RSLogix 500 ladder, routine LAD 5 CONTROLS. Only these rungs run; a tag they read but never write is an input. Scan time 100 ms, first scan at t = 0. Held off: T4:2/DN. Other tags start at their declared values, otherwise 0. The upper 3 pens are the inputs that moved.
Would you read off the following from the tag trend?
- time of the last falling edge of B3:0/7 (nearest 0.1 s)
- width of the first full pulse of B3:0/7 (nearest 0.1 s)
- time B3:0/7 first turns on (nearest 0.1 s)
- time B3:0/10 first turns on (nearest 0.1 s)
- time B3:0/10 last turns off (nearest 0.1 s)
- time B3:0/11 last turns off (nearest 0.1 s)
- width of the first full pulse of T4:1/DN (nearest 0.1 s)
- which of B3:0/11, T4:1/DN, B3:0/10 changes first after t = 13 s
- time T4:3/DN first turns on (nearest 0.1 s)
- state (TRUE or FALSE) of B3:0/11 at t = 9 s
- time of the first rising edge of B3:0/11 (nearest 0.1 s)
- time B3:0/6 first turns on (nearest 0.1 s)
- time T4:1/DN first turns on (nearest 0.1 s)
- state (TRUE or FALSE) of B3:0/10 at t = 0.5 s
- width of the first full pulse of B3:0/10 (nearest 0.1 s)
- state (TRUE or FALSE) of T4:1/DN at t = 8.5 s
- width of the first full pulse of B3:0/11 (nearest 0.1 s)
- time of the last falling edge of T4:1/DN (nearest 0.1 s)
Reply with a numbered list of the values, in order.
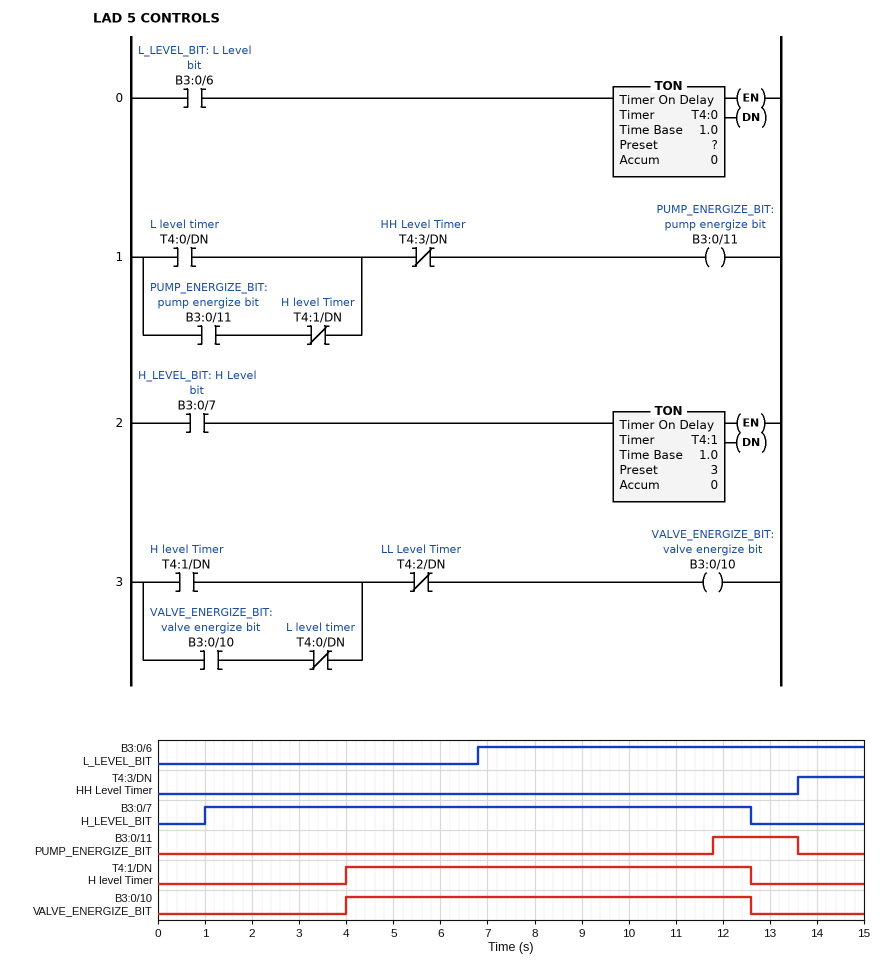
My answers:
1. 12.6 s
2. 11.6 s
3. 1.0 s
4. 4.0 s
5. 12.6 s
6. 13.6 s
7. 8.6 s
8. B3:0/11
9. 13.6 s
10. FALSE
11. 11.8 s
12. 6.8 s
13. 4.0 s
14. FALSE
15. 8.6 s
16. TRUE
17. 1.8 s
18. 12.6 s
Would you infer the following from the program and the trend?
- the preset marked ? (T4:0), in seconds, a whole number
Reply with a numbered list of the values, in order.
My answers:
1. 5 s
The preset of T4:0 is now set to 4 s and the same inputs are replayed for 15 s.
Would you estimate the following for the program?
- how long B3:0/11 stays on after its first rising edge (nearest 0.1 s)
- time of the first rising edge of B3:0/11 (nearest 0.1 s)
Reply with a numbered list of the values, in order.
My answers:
1. 2.8 s
2. 10.8 s
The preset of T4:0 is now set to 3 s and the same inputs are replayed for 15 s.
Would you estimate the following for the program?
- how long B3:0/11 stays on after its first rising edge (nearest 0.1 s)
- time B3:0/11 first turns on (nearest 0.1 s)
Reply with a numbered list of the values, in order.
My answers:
1. 3.8 s
2. 9.8 s
